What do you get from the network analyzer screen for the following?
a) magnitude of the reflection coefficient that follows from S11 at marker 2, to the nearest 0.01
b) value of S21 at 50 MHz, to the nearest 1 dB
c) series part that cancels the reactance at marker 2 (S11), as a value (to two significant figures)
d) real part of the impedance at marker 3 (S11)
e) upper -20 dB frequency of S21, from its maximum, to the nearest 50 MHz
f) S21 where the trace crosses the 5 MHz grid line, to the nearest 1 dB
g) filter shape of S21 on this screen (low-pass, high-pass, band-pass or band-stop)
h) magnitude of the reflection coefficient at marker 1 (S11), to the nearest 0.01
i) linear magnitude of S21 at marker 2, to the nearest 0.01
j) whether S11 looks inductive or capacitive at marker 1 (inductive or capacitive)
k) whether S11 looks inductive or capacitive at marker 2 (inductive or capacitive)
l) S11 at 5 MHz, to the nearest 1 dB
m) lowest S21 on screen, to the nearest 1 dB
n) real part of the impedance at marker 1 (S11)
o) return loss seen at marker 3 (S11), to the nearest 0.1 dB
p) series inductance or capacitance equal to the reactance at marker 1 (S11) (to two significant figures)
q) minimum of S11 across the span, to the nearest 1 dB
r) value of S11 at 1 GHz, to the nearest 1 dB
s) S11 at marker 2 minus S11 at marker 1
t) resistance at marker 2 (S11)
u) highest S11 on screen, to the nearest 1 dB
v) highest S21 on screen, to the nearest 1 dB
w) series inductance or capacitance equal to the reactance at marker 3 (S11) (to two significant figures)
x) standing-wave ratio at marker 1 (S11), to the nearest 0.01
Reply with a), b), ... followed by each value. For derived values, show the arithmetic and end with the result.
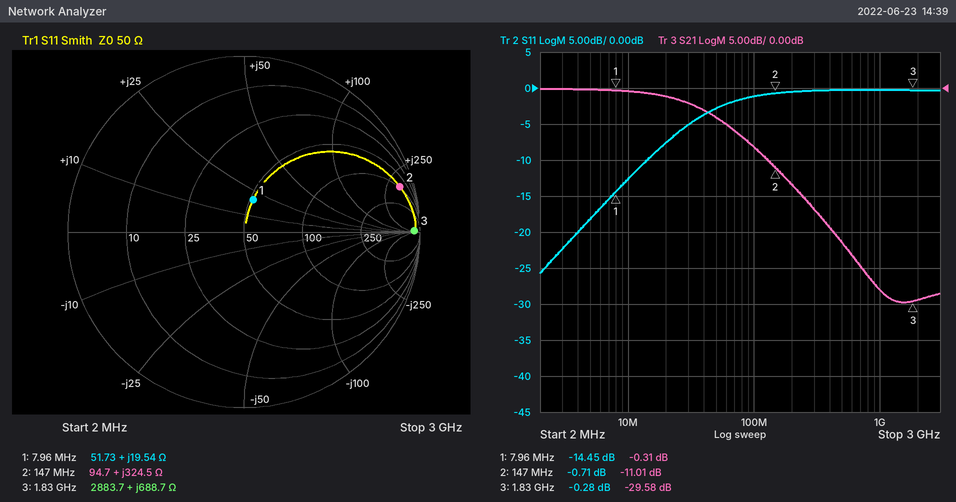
a) 10^(-0.71/20) ≈ 0.92
b) -4 dB
c) C = 1/(2π × 147 MHz × 324.5 Ω) ≈ 3.3 pF
d) 2883.7 Ω
e) 450 MHz
f) 0 dB
g) low-pass
h) 10^(-14.45/20) ≈ 0.19
i) 10^(-11.01/20) ≈ 0.28
j) inductive
k) inductive
l) -18 dB
m) -30 dB
n) 51.73 Ω
o) 0.3 dB
p) L = 19.54 Ω/(2π × 7.96 MHz) ≈ 391 nH, so 390 nH to two significant figures
q) -26 dB
r) 0 dB
s) -0.71 − (-14.45) = 13.74 dB
t) 94.7 Ω
u) 0 dB
v) 0 dB
w) L = 688.7 Ω/(2π × 1.83 GHz) ≈ 60 nH
x) 1.47
